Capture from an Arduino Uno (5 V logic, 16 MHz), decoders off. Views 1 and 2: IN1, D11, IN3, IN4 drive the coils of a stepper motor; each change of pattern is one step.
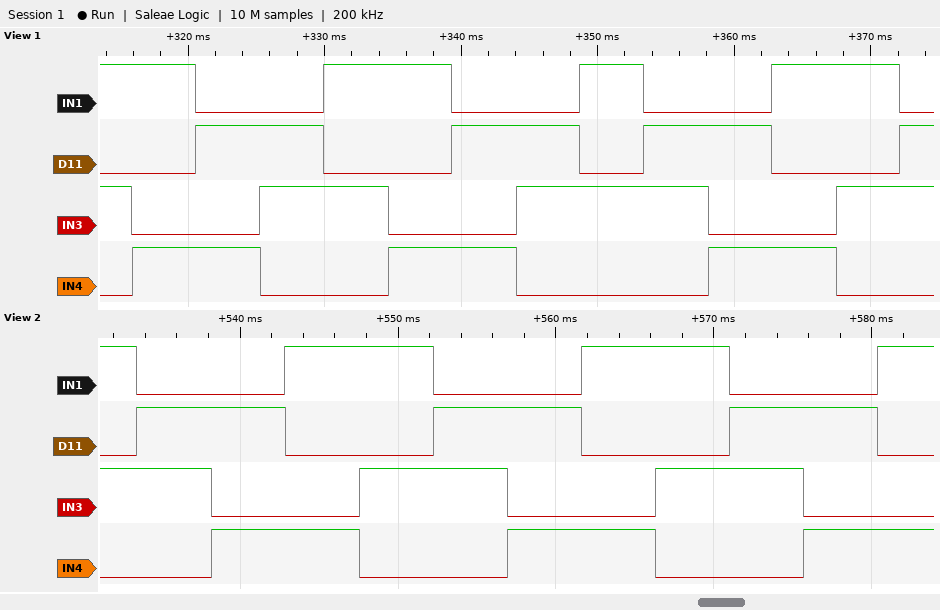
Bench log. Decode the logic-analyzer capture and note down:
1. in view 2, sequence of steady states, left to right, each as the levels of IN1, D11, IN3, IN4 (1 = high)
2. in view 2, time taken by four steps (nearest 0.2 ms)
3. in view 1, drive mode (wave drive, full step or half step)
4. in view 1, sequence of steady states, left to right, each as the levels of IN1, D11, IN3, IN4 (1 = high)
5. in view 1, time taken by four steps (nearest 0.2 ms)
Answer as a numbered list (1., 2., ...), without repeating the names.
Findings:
1. 1010 0110 0101 1001 1010 0110 0101 1001 1010 0110 0101 1001
2. 18.8 ms
3. full step
4. 1010 1001 0101 0110 1010 1001 0101 0110 1010 0110 0101 1001 1010 0110
5. 18.8 ms
